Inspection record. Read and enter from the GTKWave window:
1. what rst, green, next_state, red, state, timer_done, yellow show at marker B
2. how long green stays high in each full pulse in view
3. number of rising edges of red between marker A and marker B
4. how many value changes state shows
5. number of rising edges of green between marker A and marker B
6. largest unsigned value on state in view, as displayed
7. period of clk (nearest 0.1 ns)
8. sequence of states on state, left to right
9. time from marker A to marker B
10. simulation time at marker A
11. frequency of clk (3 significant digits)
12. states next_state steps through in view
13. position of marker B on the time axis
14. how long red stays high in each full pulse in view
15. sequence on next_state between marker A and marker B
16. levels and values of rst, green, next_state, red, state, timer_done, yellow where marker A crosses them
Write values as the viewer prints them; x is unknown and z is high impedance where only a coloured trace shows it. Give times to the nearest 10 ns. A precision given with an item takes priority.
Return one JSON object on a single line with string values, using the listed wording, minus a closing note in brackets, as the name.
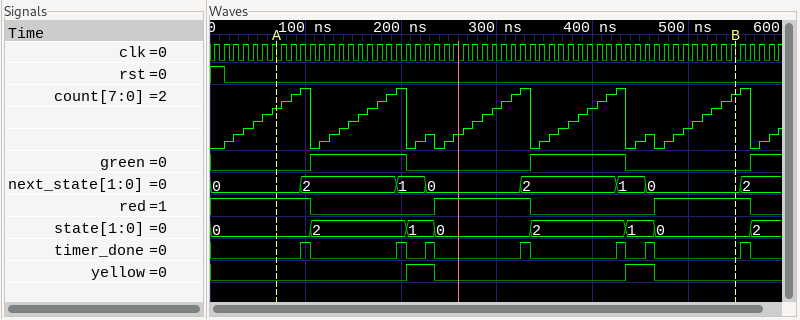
{"what rst, green, next_state, red, state, timer_done, yellow show at marker B": "rst=0, green=0, next_state=0, red=1, state=0, timer_done=0, yellow=0", "how long green stays high in each full pulse in view": "100 ns, 100 ns", "number of rising edges of red between marker A and marker B": "2", "how many value changes state shows": "7", "number of rising edges of green between marker A and marker B": "2", "largest unsigned value on state in view, as displayed": "2", "period of clk": "10 ns", "sequence of states on state, left to right": "0, 2, 1, 0, 2, 1, 0, 2", "time from marker A to marker B": "480 ns", "simulation time at marker A": "70 ns", "frequency of clk": "100 MHz", "states next_state steps through in view": "0, 2, 1, 0, 2, 1, 0, 2", "position of marker B on the time axis": "550 ns", "how long red stays high in each full pulse in view": "100 ns, 100 ns", "sequence on next_state between marker A and marker B": "0, 2, 1, 0, 2, 1, 0", "levels and values of rst, green, next_state, red, state, timer_done, yellow where marker A crosses them": "rst=0, green=0, next_state=0, red=1, state=0, timer_done=0, yellow=0"}
